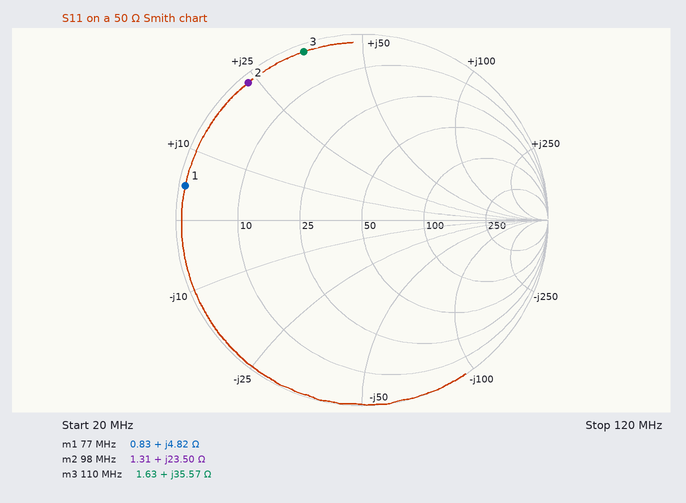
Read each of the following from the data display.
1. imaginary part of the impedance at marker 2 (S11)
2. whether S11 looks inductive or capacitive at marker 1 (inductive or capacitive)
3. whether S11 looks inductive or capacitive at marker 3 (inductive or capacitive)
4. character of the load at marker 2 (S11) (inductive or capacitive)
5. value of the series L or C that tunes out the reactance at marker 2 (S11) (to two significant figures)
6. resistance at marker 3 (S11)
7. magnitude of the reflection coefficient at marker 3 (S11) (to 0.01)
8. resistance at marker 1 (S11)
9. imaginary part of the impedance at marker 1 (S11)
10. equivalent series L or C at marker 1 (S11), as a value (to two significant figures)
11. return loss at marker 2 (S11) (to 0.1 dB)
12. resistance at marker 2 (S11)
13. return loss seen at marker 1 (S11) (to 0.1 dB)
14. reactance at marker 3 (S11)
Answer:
+23.50 Ω
inductive
inductive
inductive
69 pF
1.63 Ω
0.96
0.83 Ω
+4.82 Ω
10.0 nH
0.4 dB
1.31 Ω
0.3 dB
+35.57 Ω
